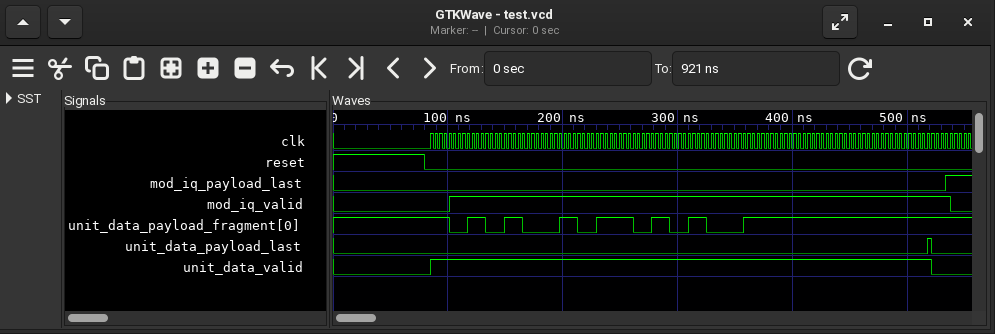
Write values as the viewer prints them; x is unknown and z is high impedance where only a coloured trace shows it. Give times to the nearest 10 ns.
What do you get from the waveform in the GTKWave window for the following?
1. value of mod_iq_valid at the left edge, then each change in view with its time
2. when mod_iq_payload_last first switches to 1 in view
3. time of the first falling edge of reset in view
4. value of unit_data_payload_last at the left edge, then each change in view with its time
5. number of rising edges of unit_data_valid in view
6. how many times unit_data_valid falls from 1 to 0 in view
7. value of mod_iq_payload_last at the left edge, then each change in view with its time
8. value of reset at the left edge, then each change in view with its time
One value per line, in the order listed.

0, 1 at 100 ns, 0 at 540 ns
530 ns
80 ns
0, 1 at 520 ns, 0 at 520 ns
1
1
0, 1 at 530 ns
1, 0 at 80 ns
